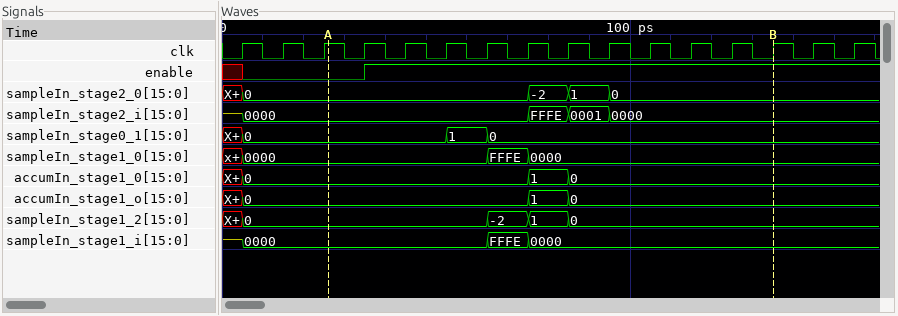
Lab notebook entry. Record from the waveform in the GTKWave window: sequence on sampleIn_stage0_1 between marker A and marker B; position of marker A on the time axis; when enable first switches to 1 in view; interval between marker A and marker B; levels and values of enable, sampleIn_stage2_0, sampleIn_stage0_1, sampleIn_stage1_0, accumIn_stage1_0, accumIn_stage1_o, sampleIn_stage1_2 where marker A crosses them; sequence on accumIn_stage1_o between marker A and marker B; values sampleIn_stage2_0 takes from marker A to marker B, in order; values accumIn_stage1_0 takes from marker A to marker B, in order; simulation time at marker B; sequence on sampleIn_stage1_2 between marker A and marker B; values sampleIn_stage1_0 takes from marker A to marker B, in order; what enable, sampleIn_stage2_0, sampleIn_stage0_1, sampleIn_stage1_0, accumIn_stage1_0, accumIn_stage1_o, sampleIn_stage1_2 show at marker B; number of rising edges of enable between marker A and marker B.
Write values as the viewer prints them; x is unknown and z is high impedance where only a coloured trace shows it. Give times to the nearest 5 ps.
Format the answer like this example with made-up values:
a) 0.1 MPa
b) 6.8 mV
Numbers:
a) 0, 1, 0
b) 25 ps
c) 35 ps
d) 110 ps
e) enable=0, sampleIn_stage2_0=0, sampleIn_stage0_1=0, sampleIn_stage1_0=0000, accumIn_stage1_0=0, accumIn_stage1_o=0, sampleIn_stage1_2=0
f) 0, 1, 0
g) 0, -2, 1, 0
h) 0, 1, 0
i) 135 ps
j) 0, -2, 1, 0
k) 0000, FFFE, 0000
l) enable=1, sampleIn_stage2_0=0, sampleIn_stage0_1=0, sampleIn_stage1_0=0000, accumIn_stage1_0=0, accumIn_stage1_o=0, sampleIn_stage1_2=0
m) 1
